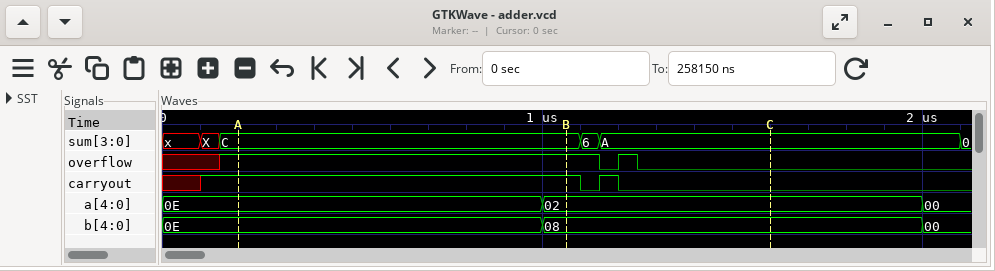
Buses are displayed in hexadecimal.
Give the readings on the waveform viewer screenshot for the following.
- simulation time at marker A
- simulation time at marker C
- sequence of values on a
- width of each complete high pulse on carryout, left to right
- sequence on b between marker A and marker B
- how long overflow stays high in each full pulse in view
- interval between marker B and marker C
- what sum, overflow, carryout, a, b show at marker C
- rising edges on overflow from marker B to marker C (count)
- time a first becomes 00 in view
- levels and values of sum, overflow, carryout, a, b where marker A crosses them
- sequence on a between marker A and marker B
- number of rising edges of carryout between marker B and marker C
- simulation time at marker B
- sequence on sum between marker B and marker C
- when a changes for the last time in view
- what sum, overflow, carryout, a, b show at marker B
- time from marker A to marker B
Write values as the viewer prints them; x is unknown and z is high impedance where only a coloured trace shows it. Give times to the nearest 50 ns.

200 ns
1600 ns
0E, 02, 00
50 ns
0E, 08
50 ns
550 ns
sum=A, overflow=0, carryout=0, a=02, b=08
1
2000 ns
sum=C, overflow=1, carryout=1, a=0E, b=0E
0E, 02
1
1050 ns
C, 6, A
2000 ns
sum=C, overflow=1, carryout=1, a=02, b=08
850 ns
